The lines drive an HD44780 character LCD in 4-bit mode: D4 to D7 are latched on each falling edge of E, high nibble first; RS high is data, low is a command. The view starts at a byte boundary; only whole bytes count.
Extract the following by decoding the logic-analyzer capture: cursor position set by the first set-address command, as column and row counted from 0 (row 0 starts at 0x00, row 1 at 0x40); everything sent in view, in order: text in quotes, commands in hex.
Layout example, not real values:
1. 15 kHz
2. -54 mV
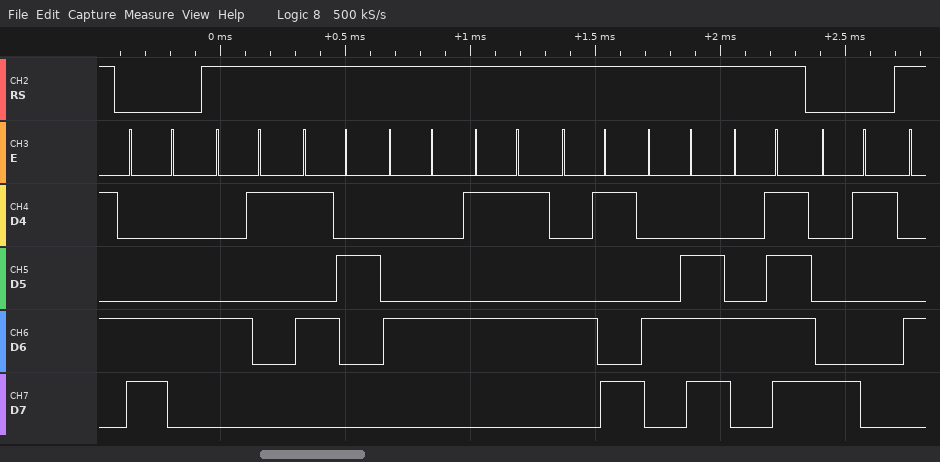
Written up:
1. column 4, row 1
2. 0xC4 "ARDUINO" 0x81
